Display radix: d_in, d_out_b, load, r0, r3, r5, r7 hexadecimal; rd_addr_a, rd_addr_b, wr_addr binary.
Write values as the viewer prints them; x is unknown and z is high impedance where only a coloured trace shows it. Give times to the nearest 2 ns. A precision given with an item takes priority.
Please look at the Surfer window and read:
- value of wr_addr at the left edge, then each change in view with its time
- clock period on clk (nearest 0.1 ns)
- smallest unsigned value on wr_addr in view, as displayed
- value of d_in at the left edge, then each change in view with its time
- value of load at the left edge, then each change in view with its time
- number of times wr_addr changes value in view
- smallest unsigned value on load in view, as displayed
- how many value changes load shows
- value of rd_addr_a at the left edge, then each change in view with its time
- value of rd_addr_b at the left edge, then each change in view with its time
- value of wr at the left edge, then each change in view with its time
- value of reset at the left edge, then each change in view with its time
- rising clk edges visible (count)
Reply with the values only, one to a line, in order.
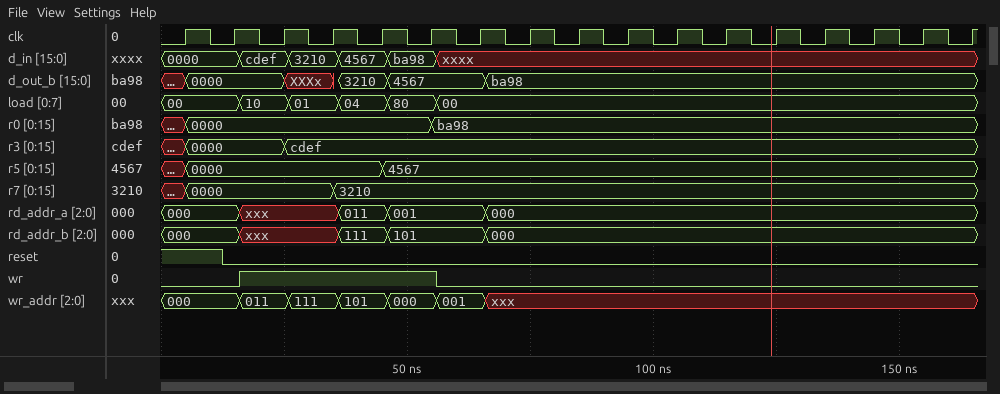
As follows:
000, 011 at 16 ns, 111 at 26 ns, 101 at 36 ns, 000 at 46 ns, 001 at 56 ns, xxx at 66 ns
10 ns
000
0000, cdef at 16 ns, 3210 at 26 ns, 4567 at 36 ns, ba98 at 46 ns, xxxx at 56 ns
00, 10 at 16 ns, 01 at 26 ns, 04 at 36 ns, 80 at 46 ns, 00 at 56 ns
6
00
5
000, xxx at 16 ns, 011 at 36 ns, 001 at 46 ns, 000 at 66 ns
000, xxx at 16 ns, 111 at 36 ns, 101 at 46 ns, 000 at 66 ns
0, 1 at 16 ns, 0 at 56 ns
1, 0 at 12 ns
17
